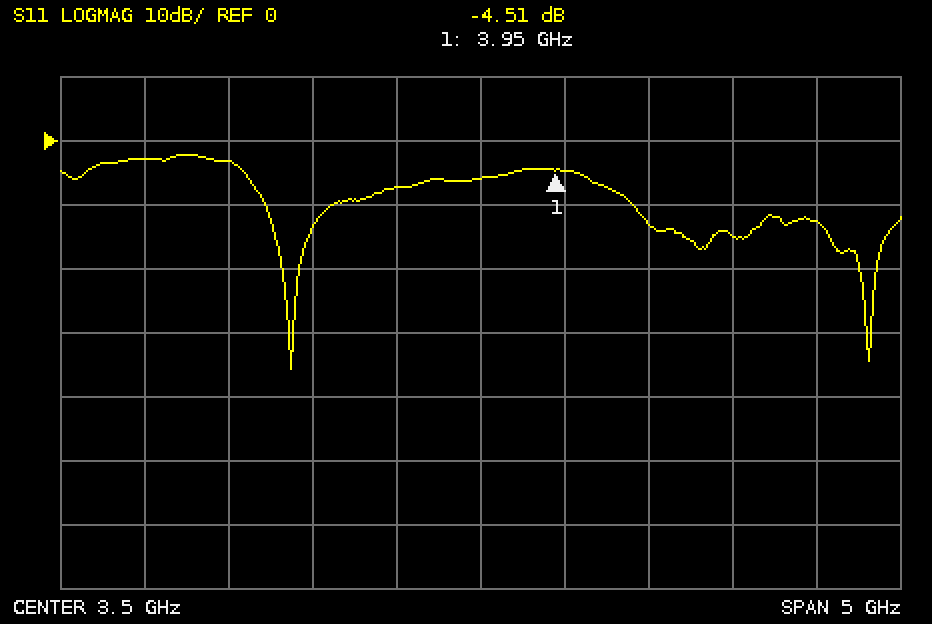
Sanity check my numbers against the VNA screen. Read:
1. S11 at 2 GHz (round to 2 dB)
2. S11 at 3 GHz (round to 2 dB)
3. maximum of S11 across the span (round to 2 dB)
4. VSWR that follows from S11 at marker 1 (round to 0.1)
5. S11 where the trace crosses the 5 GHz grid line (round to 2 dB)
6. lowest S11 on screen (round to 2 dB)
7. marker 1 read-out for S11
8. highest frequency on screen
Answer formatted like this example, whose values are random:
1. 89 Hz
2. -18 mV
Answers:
1. -4 dB
2. -8 dB
3. -2 dB
4. 3.9
5. -14 dB
6. -36 dB
7. -4.51 dB
8. 6 GHz
